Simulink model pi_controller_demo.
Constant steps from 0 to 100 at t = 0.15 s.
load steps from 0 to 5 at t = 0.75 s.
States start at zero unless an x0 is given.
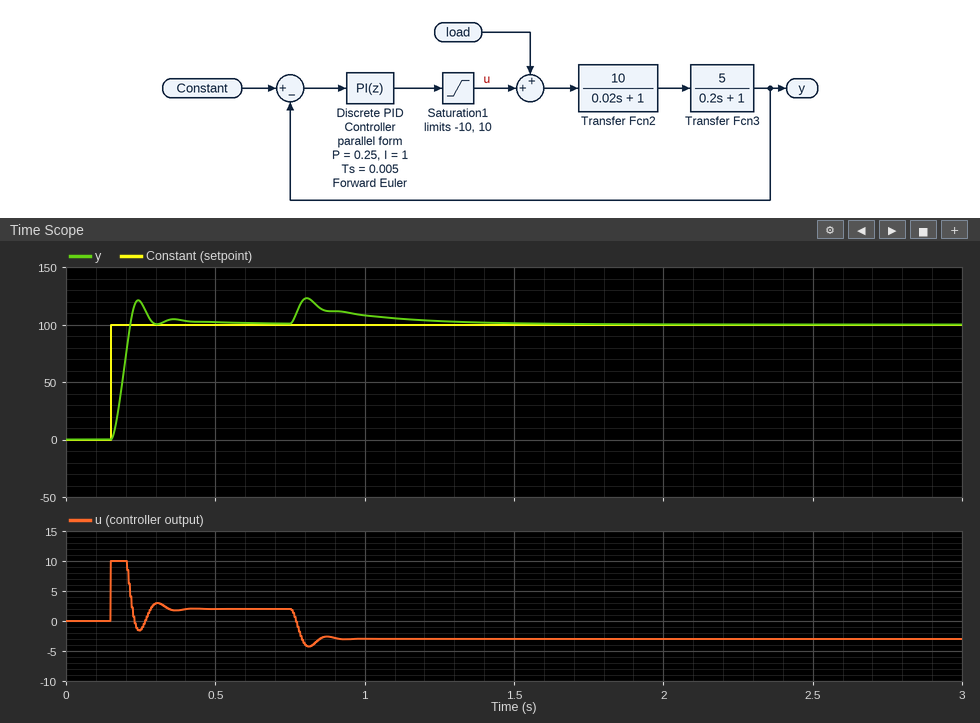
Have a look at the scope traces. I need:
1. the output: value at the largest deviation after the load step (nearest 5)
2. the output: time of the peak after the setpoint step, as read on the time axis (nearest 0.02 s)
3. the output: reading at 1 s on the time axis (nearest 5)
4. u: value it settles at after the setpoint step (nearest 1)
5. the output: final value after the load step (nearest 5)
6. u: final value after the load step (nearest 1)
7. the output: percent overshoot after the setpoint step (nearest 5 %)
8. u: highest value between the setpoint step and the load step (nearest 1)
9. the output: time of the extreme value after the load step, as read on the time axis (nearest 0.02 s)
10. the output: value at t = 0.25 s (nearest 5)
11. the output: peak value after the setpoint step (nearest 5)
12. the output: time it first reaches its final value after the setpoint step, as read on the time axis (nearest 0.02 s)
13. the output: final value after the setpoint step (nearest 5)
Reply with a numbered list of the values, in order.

1. 125
2. 0.24 s
3. 110
4. 2
5. 100
6. -3
7. 20 %
8. 10
9. 0.80 s
10. 120
11. 120
12. 0.22 s
13. 100
